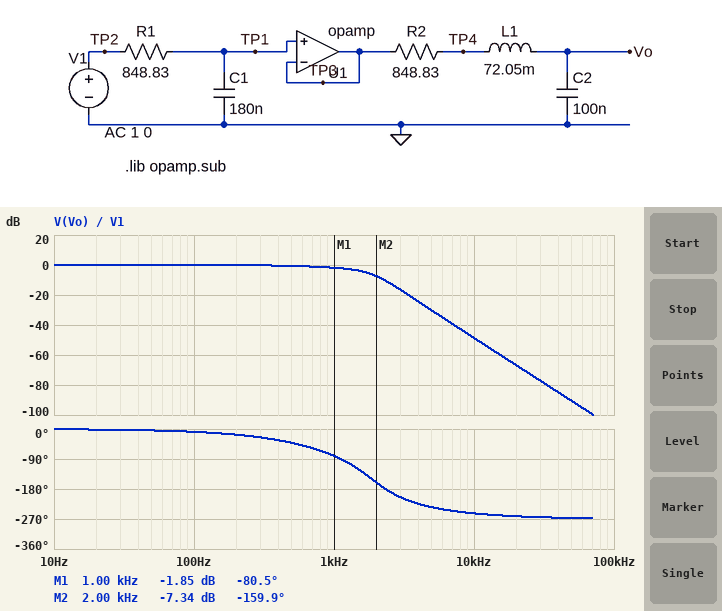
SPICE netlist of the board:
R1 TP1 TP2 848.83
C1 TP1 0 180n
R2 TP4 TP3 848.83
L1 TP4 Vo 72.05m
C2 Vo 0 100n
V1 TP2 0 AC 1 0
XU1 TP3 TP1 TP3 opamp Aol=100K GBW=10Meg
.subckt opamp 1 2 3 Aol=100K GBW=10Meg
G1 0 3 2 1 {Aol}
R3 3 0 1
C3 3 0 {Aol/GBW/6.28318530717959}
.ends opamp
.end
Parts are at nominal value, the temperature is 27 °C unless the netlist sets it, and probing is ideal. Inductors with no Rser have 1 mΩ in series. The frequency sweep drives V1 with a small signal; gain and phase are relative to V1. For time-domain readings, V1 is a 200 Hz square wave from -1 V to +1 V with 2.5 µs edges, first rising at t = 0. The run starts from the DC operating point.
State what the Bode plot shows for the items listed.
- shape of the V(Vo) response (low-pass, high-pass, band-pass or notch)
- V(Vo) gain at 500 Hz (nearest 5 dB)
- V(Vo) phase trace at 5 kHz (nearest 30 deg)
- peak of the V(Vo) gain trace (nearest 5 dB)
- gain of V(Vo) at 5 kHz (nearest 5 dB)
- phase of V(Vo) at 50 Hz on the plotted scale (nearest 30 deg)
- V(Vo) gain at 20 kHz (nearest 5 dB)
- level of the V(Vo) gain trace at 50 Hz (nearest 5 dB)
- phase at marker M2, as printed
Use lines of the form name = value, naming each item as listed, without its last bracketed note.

shape of the V(Vo) response = low-pass
V(Vo) gain at 500 Hz = 0 dB
V(Vo) phase trace at 5 kHz = -240 deg
peak of the V(Vo) gain trace = 0 dB
gain of V(Vo) at 5 kHz = -30 dB
phase of V(Vo) at 50 Hz on the plotted scale = 0 deg
V(Vo) gain at 20 kHz = -65 dB
level of the V(Vo) gain trace at 50 Hz = 0 dB
phase at marker M2, as printed = -159.9 deg
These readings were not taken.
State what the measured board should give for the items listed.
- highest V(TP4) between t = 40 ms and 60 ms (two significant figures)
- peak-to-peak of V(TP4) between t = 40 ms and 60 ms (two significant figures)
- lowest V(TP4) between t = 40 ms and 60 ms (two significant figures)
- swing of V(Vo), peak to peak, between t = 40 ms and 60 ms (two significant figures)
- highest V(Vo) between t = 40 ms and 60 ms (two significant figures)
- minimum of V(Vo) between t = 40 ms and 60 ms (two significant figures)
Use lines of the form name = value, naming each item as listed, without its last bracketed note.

highest V(TP4) between t = 40 ms and 60 ms = 1.0 V
peak-to-peak of V(TP4) between t = 40 ms and 60 ms = 2.0 V
lowest V(TP4) between t = 40 ms and 60 ms = -1.0 V
swing of V(Vo), peak to peak, between t = 40 ms and 60 ms = 2.0 V
highest V(Vo) between t = 40 ms and 60 ms = 1.0 V
minimum of V(Vo) between t = 40 ms and 60 ms = -1.0 V
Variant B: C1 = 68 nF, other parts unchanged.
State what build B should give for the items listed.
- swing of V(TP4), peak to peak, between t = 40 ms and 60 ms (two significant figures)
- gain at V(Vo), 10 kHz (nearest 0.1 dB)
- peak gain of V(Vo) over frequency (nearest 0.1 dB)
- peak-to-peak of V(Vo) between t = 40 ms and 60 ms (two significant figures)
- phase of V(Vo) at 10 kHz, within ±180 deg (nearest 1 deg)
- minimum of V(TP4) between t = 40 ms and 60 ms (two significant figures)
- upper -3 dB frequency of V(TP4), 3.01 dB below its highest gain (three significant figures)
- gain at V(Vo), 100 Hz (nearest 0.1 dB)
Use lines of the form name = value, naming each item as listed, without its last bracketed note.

swing of V(TP4), peak to peak, between t = 40 ms and 60 ms = 2.3 V
gain at V(Vo), 10 kHz = -40.4 dB
peak gain of V(Vo) over frequency = 0.5 dB
peak-to-peak of V(Vo) between t = 40 ms and 60 ms = 2.5 V
phase of V(Vo) at 10 kHz, within ±180 deg = 116 deg
minimum of V(TP4) between t = 40 ms and 60 ms = -1.1 V
upper -3 dB frequency of V(TP4), 3.01 dB below its highest gain = 1.08 kHz
gain at V(Vo), 100 Hz = 0 dB
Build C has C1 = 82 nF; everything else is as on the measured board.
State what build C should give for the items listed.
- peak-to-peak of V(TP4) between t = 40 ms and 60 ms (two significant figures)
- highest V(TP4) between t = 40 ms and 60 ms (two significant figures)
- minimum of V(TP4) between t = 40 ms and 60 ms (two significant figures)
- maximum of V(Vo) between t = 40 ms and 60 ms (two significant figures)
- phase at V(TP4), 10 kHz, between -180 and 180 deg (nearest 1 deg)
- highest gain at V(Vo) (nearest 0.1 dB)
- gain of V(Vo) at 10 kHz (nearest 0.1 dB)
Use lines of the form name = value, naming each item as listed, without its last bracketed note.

peak-to-peak of V(TP4) between t = 40 ms and 60 ms = 2.2 V
highest V(TP4) between t = 40 ms and 60 ms = 1.1 V
minimum of V(TP4) between t = 40 ms and 60 ms = -1.1 V
maximum of V(Vo) between t = 40 ms and 60 ms = 1.2 V
phase at V(TP4), 10 kHz, between -180 and 180 deg = -66 deg
highest gain at V(Vo) = 0.2 dB
gain of V(Vo) at 10 kHz = -42.0 dB
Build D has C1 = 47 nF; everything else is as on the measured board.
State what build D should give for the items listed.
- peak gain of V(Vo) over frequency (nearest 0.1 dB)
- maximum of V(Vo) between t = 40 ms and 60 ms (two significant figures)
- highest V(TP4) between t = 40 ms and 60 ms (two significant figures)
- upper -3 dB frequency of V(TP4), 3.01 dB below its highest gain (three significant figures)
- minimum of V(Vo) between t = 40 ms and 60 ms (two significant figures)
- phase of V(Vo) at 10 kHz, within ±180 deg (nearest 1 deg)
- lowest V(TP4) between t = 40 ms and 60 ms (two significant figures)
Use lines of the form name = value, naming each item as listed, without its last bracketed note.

peak gain of V(Vo) over frequency = 0.8 dB
maximum of V(Vo) between t = 40 ms and 60 ms = 1.3 V
highest V(TP4) between t = 40 ms and 60 ms = 1.2 V
upper -3 dB frequency of V(TP4), 3.01 dB below its highest gain = 1.12 kHz
minimum of V(Vo) between t = 40 ms and 60 ms = -1.3 V
phase of V(Vo) at 10 kHz, within ±180 deg = 123 deg
lowest V(TP4) between t = 40 ms and 60 ms = -1.2 V
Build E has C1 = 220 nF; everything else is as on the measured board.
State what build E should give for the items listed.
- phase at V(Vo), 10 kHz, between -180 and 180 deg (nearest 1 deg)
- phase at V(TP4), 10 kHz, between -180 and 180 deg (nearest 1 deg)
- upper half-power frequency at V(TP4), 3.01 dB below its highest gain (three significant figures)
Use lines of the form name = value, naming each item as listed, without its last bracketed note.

phase at V(Vo), 10 kHz, between -180 and 180 deg = 106 deg
phase at V(TP4), 10 kHz, between -180 and 180 deg = -74 deg
upper half-power frequency at V(TP4), 3.01 dB below its highest gain = 703 Hz
